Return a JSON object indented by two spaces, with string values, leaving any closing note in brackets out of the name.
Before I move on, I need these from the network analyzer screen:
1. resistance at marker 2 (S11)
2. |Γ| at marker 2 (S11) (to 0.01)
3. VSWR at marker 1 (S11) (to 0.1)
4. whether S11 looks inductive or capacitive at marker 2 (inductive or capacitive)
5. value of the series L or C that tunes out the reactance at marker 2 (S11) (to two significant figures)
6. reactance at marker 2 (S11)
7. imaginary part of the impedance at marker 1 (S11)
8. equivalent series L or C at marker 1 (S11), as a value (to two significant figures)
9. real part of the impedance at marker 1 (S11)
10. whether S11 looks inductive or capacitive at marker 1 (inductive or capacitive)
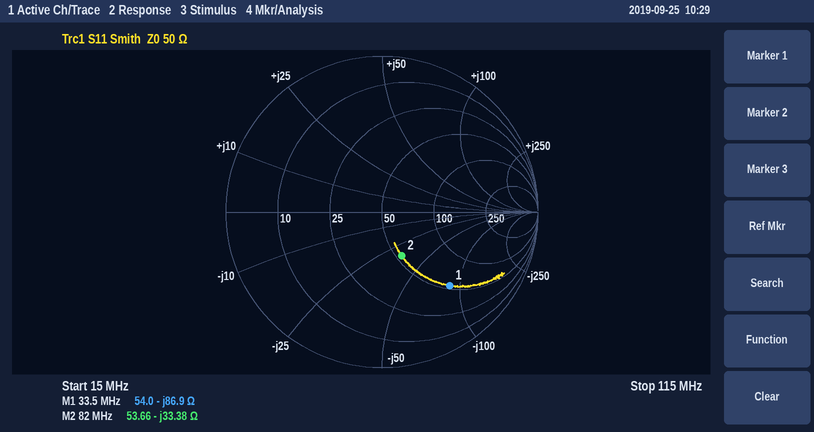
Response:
{
  "resistance at marker 2": "53.66 Ω",
  "|Γ| at marker 2 (S11)": "0.31",
  "VSWR at marker 1 (S11)": "4.6",
  "whether S11 looks inductive or capacitive at marker 2": "capacitive",
  "value of the series L or C that tunes out the reactance at marker 2 (S11)": "65 nH",
  "reactance at marker 2": "-33.38 Ω",
  "imaginary part of the impedance at marker 1": "-86.9 Ω",
  "equivalent series L or C at marker 1 (S11), as a value": "55 pF",
  "real part of the impedance at marker 1": "54.0 Ω",
  "whether S11 looks inductive or capacitive at marker 1": "capacitive"
}
